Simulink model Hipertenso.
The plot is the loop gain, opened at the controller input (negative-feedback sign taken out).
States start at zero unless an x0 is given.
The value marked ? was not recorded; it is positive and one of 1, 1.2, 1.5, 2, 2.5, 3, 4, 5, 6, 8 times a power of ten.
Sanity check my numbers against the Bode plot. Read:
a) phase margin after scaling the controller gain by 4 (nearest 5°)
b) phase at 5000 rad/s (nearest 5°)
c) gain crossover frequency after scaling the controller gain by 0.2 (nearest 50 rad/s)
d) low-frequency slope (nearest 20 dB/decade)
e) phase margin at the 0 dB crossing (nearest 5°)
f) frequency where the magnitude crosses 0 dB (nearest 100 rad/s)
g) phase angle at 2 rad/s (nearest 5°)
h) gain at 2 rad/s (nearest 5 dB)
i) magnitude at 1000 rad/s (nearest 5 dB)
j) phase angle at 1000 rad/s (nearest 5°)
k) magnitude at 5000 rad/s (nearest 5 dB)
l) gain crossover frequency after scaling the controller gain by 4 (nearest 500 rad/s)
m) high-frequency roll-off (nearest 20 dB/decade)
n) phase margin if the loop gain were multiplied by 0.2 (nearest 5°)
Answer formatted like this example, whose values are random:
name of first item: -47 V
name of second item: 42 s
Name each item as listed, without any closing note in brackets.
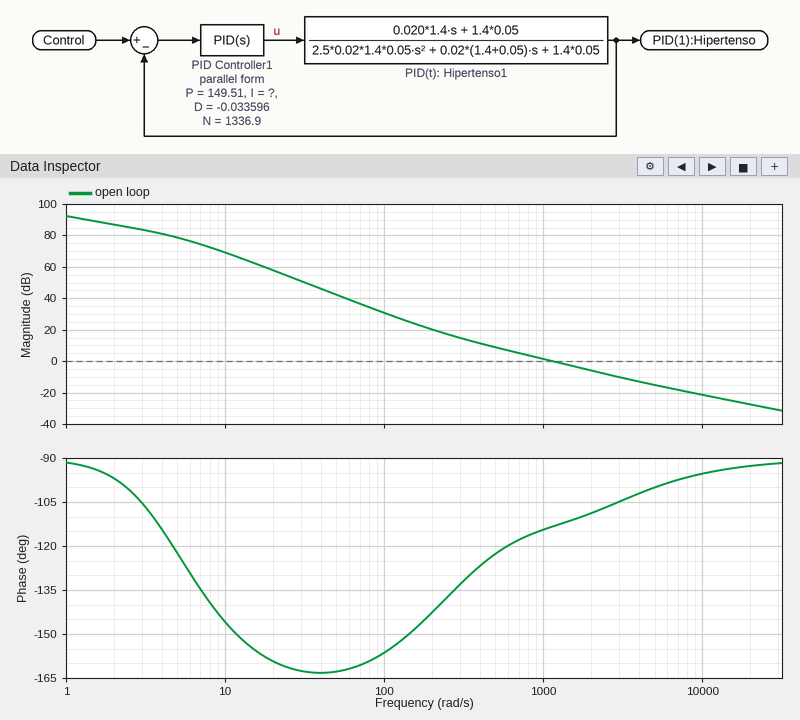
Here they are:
phase margin after scaling the controller gain by 4: 75°
phase at 5000 rad/s: -100°
gain crossover frequency after scaling the controller gain by 0.2: 300 rad/s
low-frequency slope: -20 dB/decade
phase margin at the 0 dB crossing: 65°
frequency where the magnitude crosses 0 dB: 1100 rad/s
phase angle at 2 rad/s: -95°
gain at 2 rad/s: 85 dB
magnitude at 1000 rad/s: 0 dB
phase angle at 1000 rad/s: -115°
magnitude at 5000 rad/s: -15 dB
gain crossover frequency after scaling the controller gain by 4: 3500 rad/s
high-frequency roll-off: -20 dB/decade
phase margin if the loop gain were multiplied by 0.2: 50°
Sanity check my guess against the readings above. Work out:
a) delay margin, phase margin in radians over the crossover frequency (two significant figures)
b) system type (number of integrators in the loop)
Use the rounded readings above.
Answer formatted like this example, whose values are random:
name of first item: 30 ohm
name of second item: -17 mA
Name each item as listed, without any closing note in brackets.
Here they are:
delay margin, phase margin in radians over the crossover frequency: 0.0010 s
system type: 1
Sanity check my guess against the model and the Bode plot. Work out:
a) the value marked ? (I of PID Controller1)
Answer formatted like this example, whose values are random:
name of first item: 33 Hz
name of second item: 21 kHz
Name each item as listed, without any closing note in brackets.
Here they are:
the value marked ?: 40000
